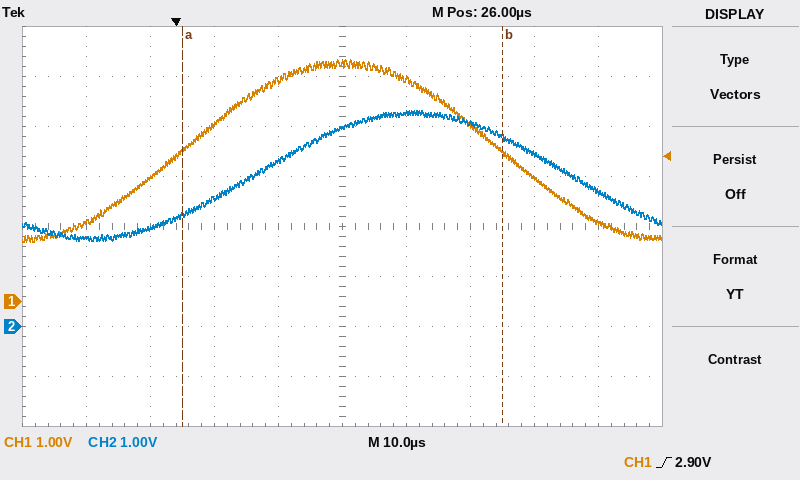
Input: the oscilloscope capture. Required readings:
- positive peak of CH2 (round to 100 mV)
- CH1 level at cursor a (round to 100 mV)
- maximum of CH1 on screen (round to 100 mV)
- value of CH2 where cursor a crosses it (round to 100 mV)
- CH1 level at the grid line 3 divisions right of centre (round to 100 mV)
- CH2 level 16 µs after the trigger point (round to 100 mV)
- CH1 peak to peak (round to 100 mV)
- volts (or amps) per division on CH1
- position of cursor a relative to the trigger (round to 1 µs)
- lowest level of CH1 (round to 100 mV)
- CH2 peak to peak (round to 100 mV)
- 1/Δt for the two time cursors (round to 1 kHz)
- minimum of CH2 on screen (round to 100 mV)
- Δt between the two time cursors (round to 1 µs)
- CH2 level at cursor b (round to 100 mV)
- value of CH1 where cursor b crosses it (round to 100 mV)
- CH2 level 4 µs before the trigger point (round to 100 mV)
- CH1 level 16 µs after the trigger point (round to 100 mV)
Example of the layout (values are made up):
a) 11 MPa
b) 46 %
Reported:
a) 4.3 V
b) 3.0 V
c) 4.8 V
d) 2.2 V
e) 2.5 V
f) 3.3 V
g) 3.6 V
h) 1 V
i) +1 µs
j) 1.2 V
k) 2.6 V
l) 20 kHz
m) 1.7 V
n) 50 µs
o) 3.8 V
p) 3.0 V
q) 2.0 V
r) 4.4 V
